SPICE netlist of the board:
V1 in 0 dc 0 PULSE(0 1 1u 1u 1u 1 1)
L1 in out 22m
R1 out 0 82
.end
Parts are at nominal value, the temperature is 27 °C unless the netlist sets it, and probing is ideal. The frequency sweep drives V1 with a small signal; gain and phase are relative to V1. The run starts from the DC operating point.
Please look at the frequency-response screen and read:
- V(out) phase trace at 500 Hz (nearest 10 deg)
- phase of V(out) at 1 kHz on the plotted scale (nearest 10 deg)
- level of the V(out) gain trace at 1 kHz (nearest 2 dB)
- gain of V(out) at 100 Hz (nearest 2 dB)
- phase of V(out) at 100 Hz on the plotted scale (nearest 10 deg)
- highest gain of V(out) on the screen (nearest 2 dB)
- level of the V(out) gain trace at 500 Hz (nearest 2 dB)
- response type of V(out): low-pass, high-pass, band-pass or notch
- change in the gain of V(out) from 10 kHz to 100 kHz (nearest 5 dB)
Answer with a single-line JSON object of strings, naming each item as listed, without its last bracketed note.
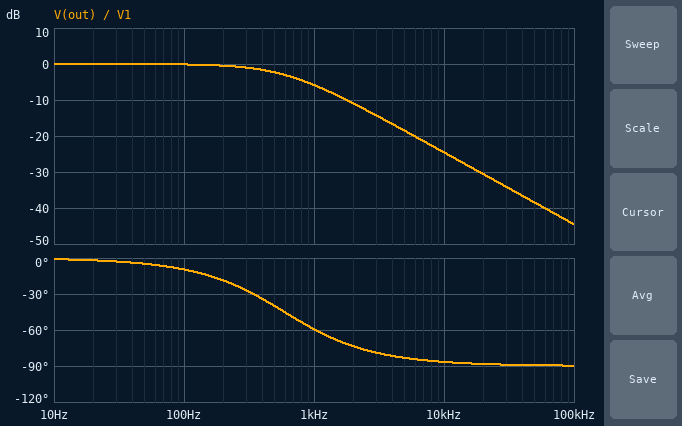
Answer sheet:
{"V(out) phase trace at 500 Hz": "-40 deg", "phase of V(out) at 1 kHz on the plotted scale": "-60 deg", "level of the V(out) gain trace at 1 kHz": "-6 dB", "gain of V(out) at 100 Hz": "0 dB", "phase of V(out) at 100 Hz on the plotted scale": "-10 deg", "highest gain of V(out) on the screen": "0 dB", "level of the V(out) gain trace at 500 Hz": "-2 dB", "response type of V(out): low-pass, high-pass, band-pass or notch": "low-pass", "change in the gain of V(out) from 10 kHz to 100 kHz": "-20 dB"}
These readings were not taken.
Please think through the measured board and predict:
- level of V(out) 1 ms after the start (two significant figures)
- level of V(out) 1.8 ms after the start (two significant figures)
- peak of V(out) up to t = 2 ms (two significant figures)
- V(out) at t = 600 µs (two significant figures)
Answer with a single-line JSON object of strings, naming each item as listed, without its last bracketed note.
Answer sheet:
{"level of V(out) 1 ms after the start": "980 mV", "level of V(out) 1.8 ms after the start": "1.0 V", "peak of V(out) up to t = 2 ms": "1.0 V", "V(out) at t = 600 µs": "890 mV"}
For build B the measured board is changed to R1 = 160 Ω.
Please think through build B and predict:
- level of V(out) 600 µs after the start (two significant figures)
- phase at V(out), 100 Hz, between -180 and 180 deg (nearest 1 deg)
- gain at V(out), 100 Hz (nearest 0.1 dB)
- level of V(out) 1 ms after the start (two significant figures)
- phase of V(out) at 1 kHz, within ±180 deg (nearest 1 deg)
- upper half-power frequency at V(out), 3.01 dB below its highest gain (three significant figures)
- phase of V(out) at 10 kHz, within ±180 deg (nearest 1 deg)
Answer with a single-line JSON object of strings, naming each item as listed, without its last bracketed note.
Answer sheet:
{"level of V(out) 600 µs after the start": "990 mV", "phase at V(out), 100 Hz, between -180 and 180 deg": "-5 deg", "gain at V(out), 100 Hz": "0 dB", "level of V(out) 1 ms after the start": "1.0 V", "phase of V(out) at 1 kHz, within ±180 deg": "-41 deg", "upper half-power frequency at V(out), 3.01 dB below its highest gain": "1.16 kHz", "phase of V(out) at 10 kHz, within ±180 deg": "-83 deg"}
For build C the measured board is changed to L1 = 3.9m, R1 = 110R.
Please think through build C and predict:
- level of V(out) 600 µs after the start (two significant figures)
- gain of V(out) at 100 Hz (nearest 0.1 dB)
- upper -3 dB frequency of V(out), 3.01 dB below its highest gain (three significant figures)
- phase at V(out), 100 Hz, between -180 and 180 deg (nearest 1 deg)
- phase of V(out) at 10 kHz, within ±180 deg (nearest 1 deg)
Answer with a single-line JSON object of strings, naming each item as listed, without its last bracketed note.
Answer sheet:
{"level of V(out) 600 µs after the start": "1.0 V", "gain of V(out) at 100 Hz": "0 dB", "upper -3 dB frequency of V(out), 3.01 dB below its highest gain": "4.49 kHz", "phase at V(out), 100 Hz, between -180 and 180 deg": "-1 deg", "phase of V(out) at 10 kHz, within ±180 deg": "-66 deg"}
